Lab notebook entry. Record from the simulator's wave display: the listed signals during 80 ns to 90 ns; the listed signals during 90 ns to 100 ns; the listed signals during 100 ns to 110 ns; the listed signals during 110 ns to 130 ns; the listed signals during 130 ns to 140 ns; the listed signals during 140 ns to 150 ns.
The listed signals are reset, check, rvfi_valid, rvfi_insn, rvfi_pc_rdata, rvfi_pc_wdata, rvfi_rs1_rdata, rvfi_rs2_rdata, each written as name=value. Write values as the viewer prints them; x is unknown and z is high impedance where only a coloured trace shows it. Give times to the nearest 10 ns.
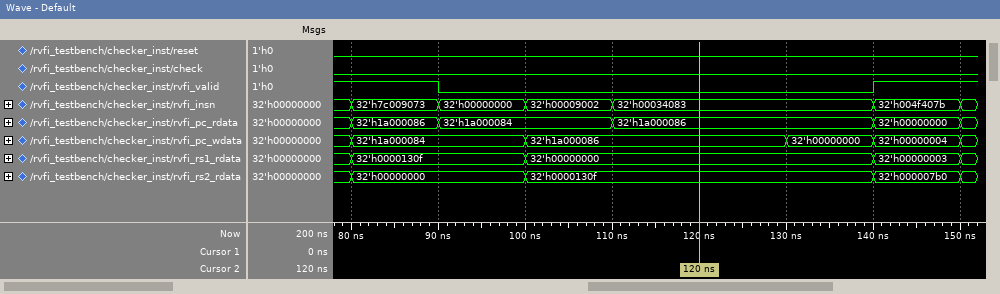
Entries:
reset=0, check=0, rvfi_valid=1, rvfi_insn=32'h7c009073, rvfi_pc_rdata=32'h1a000086, rvfi_pc_wdata=32'h1a000084, rvfi_rs1_rdata=32'h0000130f, rvfi_rs2_rdata=32'h00000000
reset=0, check=0, rvfi_valid=0, rvfi_insn=32'h00000000, rvfi_pc_rdata=32'h1a000084, rvfi_pc_wdata=32'h1a000084, rvfi_rs1_rdata=32'h0000130f, rvfi_rs2_rdata=32'h00000000
reset=0, check=0, rvfi_valid=0, rvfi_insn=32'h00009002, rvfi_pc_rdata=32'h1a000084, rvfi_pc_wdata=32'h1a000086, rvfi_rs1_rdata=32'h00000000, rvfi_rs2_rdata=32'h0000130f
reset=0, check=0, rvfi_valid=0, rvfi_insn=32'h00034083, rvfi_pc_rdata=32'h1a000086, rvfi_pc_wdata=32'h1a000086, rvfi_rs1_rdata=32'h00000000, rvfi_rs2_rdata=32'h0000130f
reset=0, check=0, rvfi_valid=0, rvfi_insn=32'h00034083, rvfi_pc_rdata=32'h1a000086, rvfi_pc_wdata=32'h00000000, rvfi_rs1_rdata=32'h00000000, rvfi_rs2_rdata=32'h0000130f
reset=0, check=0, rvfi_valid=1, rvfi_insn=32'h004f407b, rvfi_pc_rdata=32'h00000000, rvfi_pc_wdata=32'h00000004, rvfi_rs1_rdata=32'h00000003, rvfi_rs2_rdata=32'h000007b0
